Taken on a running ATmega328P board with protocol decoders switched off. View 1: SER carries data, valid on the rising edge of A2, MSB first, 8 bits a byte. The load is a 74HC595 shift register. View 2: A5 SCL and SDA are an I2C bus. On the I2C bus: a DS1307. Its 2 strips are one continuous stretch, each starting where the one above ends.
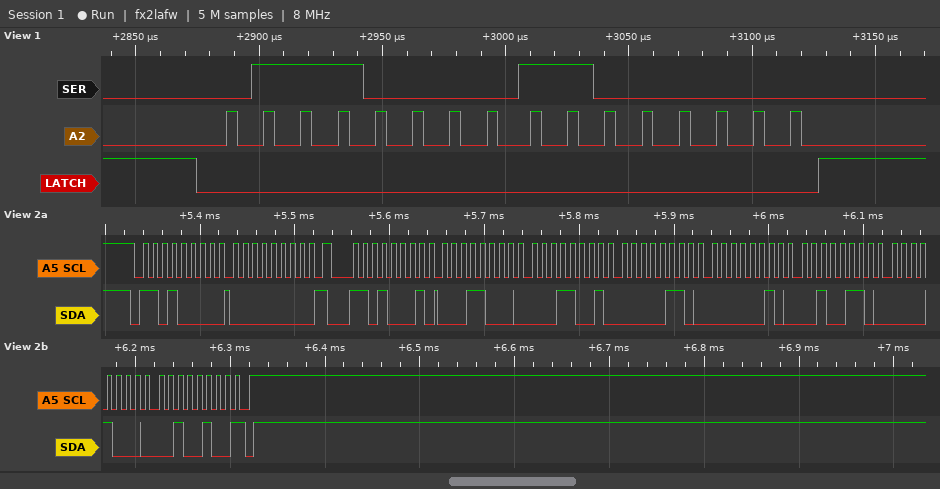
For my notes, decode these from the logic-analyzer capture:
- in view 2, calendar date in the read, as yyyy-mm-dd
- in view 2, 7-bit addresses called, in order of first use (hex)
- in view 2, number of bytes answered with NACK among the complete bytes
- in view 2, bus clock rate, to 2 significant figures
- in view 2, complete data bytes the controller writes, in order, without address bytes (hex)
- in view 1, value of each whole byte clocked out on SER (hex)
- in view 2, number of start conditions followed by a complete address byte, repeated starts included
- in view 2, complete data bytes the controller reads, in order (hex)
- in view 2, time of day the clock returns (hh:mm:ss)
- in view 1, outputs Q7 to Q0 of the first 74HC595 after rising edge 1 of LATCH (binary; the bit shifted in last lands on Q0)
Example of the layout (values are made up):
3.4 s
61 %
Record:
2024-08-26
0x68
1
100 kHz
00
0x70 0xC0
2
18 19 06 02 26 08 24
06:19:18
11000000
